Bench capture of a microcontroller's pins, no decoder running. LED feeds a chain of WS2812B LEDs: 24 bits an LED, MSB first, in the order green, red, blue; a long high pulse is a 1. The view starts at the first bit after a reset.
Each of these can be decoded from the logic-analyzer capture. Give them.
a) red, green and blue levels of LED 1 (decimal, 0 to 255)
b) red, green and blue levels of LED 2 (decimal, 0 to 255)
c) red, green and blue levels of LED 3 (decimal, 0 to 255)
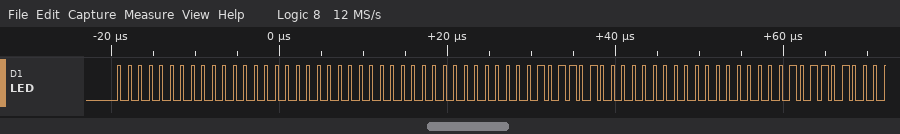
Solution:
0, 0, 0
0, 0, 180
0, 0, 180
